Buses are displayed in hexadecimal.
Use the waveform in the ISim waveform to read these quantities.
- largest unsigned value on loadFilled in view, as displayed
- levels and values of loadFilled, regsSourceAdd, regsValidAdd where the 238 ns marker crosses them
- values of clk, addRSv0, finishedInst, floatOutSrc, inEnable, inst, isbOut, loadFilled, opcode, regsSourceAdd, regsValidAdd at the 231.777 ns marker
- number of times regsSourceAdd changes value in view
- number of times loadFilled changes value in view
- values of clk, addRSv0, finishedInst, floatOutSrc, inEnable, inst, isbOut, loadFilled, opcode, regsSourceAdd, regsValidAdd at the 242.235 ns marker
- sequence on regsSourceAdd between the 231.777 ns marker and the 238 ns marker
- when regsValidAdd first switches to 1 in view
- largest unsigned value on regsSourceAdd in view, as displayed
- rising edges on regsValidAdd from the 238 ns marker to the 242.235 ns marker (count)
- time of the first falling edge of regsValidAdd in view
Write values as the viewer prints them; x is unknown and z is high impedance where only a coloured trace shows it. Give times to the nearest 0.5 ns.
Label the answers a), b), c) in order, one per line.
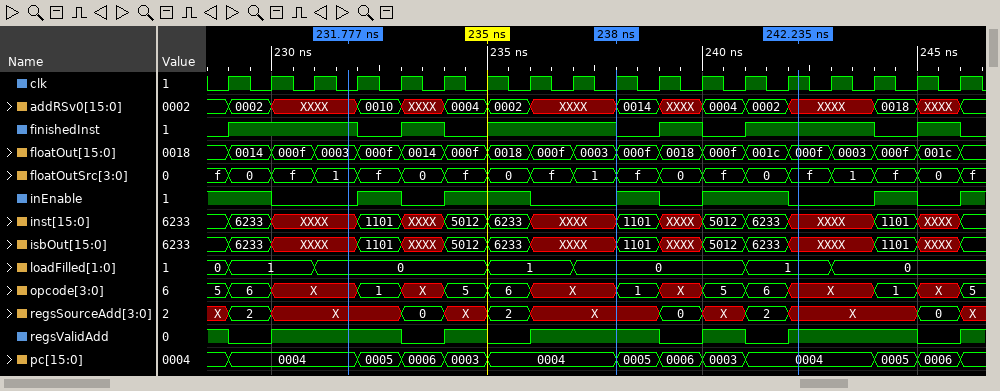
a) 1
b) loadFilled=0, regsSourceAdd=X, regsValidAdd=1
c) clk=0, addRSv0=XXXX, finishedInst=1, floatOutSrc=1, inEnable=0, inst=XXXX, isbOut=XXXX, loadFilled=0, opcode=X, regsSourceAdd=X, regsValidAdd=1
d) 12
e) 6
f) clk=1, addRSv0=XXXX, finishedInst=1, floatOutSrc=f, inEnable=0, inst=XXXX, isbOut=XXXX, loadFilled=1, opcode=X, regsSourceAdd=X, regsValidAdd=1
g) X, 0, X, 2, X
h) 230 ns
i) 2
j) 2
k) 229 ns
